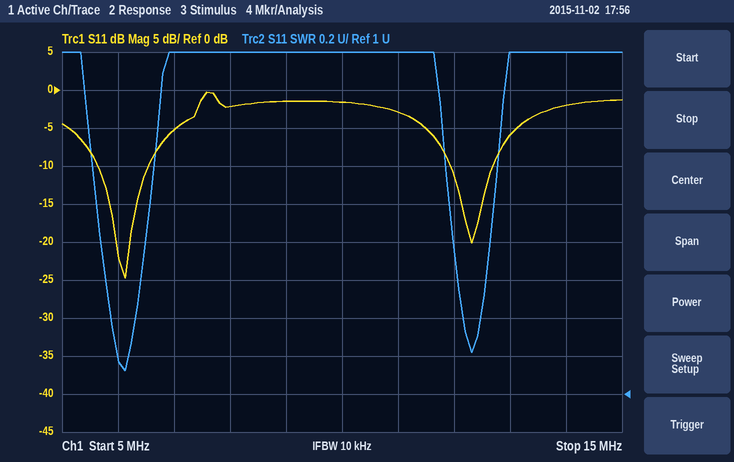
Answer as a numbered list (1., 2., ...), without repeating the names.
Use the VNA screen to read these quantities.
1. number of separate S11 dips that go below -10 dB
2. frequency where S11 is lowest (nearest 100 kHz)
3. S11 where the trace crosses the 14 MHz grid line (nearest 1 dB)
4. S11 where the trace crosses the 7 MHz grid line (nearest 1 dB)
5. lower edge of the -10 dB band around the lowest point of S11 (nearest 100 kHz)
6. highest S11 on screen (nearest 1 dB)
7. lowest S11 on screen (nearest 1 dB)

1. 2
2. 6.1 MHz
3. -2 dB
4. -5 dB
5. 5.6 MHz
6. 0 dB
7. -25 dB
